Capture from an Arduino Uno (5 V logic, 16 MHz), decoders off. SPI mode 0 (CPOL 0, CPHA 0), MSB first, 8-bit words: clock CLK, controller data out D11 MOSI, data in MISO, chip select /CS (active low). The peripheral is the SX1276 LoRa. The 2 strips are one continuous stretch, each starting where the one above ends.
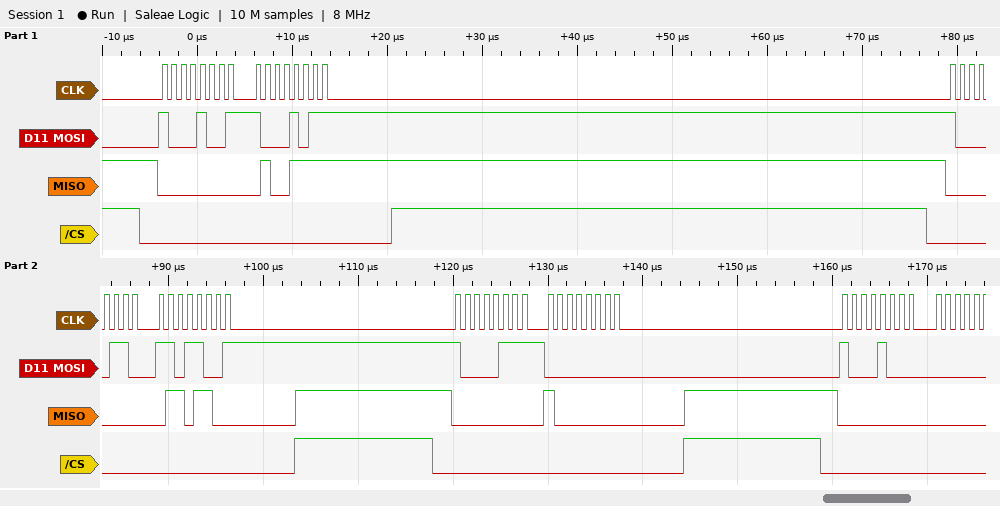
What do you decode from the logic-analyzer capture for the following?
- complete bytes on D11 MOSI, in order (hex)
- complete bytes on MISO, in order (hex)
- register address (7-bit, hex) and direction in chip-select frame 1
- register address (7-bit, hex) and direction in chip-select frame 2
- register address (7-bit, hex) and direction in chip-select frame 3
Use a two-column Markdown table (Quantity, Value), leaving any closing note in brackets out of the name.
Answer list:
| Quantity | Value |
|---|---|
| complete bytes on D11 MOSI, in order | 89 8B 86 D9 87 00 88 |
| complete bytes on MISO, in order | 00 4F 00 6C 00 80 00 |
| register address (7-bit, hex) and direction in chip-select frame 1 | 0x09 write |
| register address (7-bit, hex) and direction in chip-select frame 2 | 0x06 write |
| register address (7-bit, hex) and direction in chip-select frame 3 | 0x07 write |
